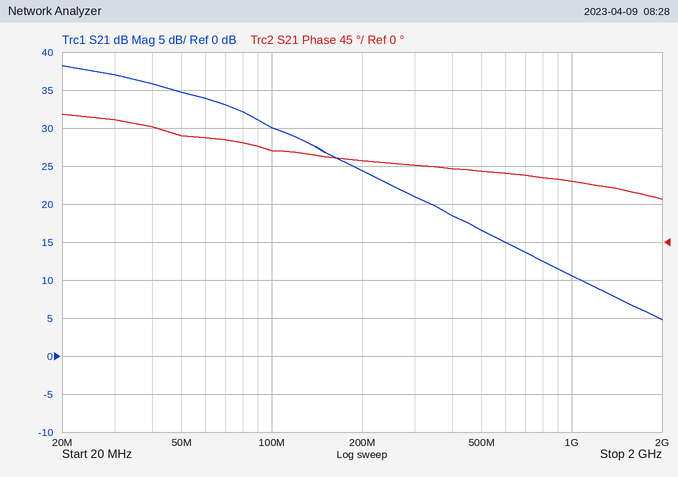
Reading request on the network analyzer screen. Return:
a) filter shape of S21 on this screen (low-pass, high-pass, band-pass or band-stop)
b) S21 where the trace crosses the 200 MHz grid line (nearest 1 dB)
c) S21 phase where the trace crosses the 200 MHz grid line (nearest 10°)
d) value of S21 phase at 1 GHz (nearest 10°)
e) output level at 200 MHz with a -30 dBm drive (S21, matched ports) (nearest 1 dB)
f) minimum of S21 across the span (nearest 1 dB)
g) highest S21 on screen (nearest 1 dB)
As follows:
low-pass
24 dB
100°
70°
-6 dBm
5 dB
38 dB
